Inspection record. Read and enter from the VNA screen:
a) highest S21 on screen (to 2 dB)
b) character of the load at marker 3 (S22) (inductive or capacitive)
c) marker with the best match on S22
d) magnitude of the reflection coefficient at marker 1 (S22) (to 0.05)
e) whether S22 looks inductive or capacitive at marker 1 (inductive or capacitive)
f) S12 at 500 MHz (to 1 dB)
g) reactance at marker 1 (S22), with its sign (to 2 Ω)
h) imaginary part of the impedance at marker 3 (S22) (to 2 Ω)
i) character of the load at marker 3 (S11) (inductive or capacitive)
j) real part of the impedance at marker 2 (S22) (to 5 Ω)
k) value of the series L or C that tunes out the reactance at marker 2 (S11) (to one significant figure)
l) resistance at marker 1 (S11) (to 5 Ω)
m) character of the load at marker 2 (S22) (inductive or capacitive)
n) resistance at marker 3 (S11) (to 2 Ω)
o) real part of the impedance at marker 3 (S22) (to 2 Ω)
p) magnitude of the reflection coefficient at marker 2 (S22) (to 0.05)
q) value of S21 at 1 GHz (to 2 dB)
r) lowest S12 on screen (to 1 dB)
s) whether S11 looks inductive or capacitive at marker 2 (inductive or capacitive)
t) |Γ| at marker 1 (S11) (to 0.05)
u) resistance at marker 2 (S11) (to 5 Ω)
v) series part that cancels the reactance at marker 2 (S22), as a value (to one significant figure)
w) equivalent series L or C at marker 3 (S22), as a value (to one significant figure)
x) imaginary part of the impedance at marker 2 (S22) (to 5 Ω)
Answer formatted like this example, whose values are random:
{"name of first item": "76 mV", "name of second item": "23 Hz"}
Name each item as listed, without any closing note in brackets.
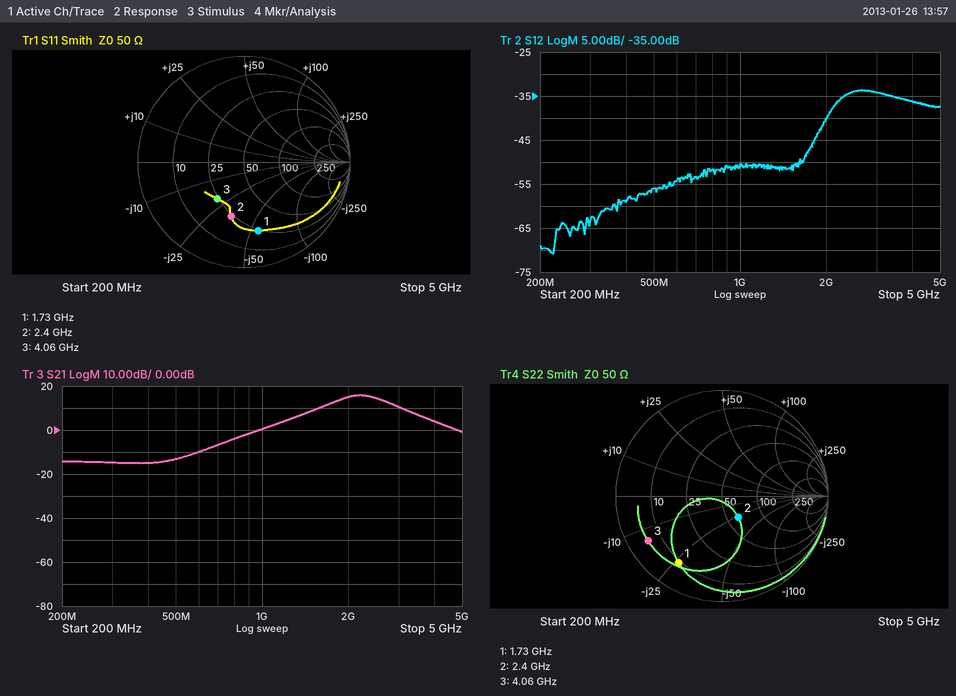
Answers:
{"highest S21 on screen": "16 dB", "character of the load at marker 3 (S22)": "capacitive", "marker with the best match on S22": "marker 2", "magnitude of the reflection coefficient at marker 1 (S22)": "0.75", "whether S22 looks inductive or capacitive at marker 1": "capacitive", "S12 at 500 MHz": "-56 dB", "reactance at marker 1 (S22), with its sign": "-26 Ω", "imaginary part of the impedance at marker 3 (S22)": "-14 Ω", "character of the load at marker 3 (S11)": "capacitive", "real part of the impedance at marker 2 (S22)": "60 Ω", "value of the series L or C that tunes out the reactance at marker 2 (S11)": "2 nH", "resistance at marker 1 (S11)": "25 Ω", "character of the load at marker 2 (S22)": "capacitive", "resistance at marker 3 (S11)": "24 Ω", "real part of the impedance at marker 3 (S22)": "6 Ω", "magnitude of the reflection coefficient at marker 2 (S22)": "0.25", "value of S21 at 1 GHz": "0 dB", "lowest S12 on screen": "-71 dB", "whether S11 looks inductive or capacitive at marker 2": "capacitive", "|Γ| at marker 1 (S11)": "0.65", "resistance at marker 2 (S11)": "25 Ω", "series part that cancels the reactance at marker 2 (S22), as a value": "2 nH", "equivalent series L or C at marker 3 (S22), as a value": "3 pF", "imaginary part of the impedance at marker 2 (S22)": "-25 Ω"}
